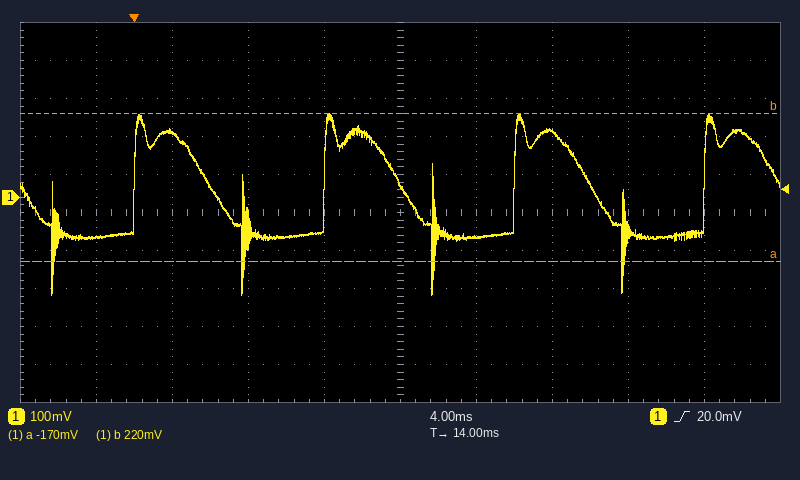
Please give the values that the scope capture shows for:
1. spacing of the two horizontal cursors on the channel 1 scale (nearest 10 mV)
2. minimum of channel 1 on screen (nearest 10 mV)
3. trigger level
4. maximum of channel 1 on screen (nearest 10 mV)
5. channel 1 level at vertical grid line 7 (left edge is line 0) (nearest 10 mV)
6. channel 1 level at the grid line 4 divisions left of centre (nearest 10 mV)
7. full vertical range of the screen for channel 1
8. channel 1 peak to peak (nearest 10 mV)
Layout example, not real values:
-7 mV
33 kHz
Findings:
390 mV
-260 mV
20.0 mV
220 mV
170 mV
-110 mV
1 V
480 mV
